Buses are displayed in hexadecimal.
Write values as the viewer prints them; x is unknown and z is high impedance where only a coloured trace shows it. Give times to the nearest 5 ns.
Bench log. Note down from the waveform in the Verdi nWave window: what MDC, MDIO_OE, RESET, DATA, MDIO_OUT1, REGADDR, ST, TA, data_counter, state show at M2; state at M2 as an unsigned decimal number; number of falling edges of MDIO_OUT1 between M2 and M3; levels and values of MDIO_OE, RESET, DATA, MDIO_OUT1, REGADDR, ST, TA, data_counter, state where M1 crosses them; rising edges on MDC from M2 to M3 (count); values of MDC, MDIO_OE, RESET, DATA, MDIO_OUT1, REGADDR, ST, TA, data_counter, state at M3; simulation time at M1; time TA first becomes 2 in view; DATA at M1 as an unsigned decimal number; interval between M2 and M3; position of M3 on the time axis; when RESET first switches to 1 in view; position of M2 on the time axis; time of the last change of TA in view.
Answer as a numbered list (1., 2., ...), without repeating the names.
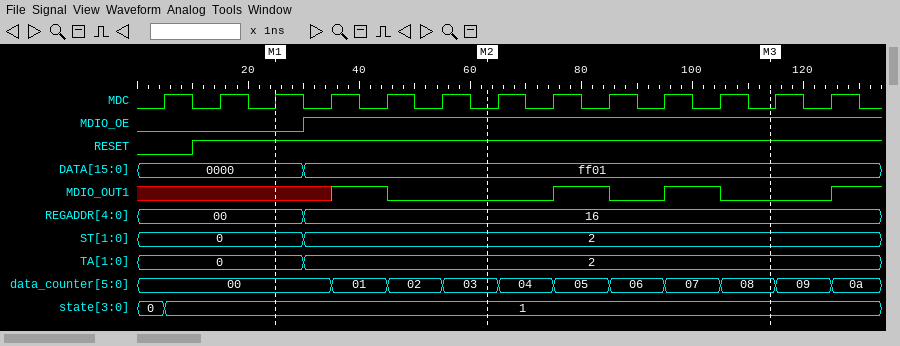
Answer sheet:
1. MDC=0, MDIO_OE=1, RESET=1, DATA=ff01, MDIO_OUT1=0, REGADDR=16, ST=2, TA=2, data_counter=03, state=1
2. 1
3. 2
4. MDIO_OE=0, RESET=1, DATA=0000, MDIO_OUT1=x, REGADDR=00, ST=0, TA=0, data_counter=00, state=1
5. 5
6. MDC=0, MDIO_OE=1, RESET=1, DATA=ff01, MDIO_OUT1=0, REGADDR=16, ST=2, TA=2, data_counter=08, state=1
7. 25 ns
8. 30 ns
9. 0
10. 50 ns
11. 115 ns
12. 10 ns
13. 65 ns
14. 30 ns
